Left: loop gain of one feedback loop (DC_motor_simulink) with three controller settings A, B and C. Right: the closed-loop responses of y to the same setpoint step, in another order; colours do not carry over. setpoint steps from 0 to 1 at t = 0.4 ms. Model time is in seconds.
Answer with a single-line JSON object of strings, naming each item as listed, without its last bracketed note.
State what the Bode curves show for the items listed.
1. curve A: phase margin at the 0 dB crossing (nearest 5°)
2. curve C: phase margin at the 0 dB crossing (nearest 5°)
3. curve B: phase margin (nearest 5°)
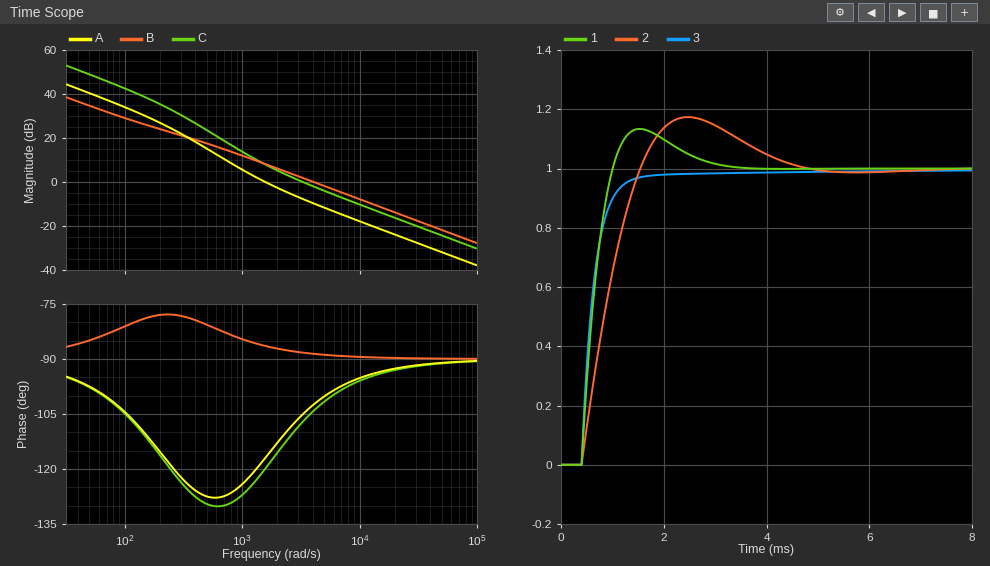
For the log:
{"curve A: phase margin at the 0 dB crossing": "65°", "curve C: phase margin at the 0 dB crossing": "75°", "curve B: phase margin": "90°"}
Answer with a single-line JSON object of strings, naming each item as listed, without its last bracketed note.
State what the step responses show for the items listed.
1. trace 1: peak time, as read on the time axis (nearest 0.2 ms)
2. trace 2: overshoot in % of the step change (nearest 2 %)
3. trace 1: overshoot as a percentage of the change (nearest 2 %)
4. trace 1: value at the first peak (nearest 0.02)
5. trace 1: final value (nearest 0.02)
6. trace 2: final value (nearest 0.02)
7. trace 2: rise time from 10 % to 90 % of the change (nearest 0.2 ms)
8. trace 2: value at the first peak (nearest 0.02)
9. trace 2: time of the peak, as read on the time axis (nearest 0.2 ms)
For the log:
{"trace 1: peak time, as read on the time axis": "1.6 ms", "trace 2: overshoot in % of the step change": "18 %", "trace 1: overshoot as a percentage of the change": "14 %", "trace 1: value at the first peak": "1.14", "trace 1: final value": "1.00", "trace 2: final value": "1.00", "trace 2: rise time from 10 % to 90 % of the change": "0.8 ms", "trace 2: value at the first peak": "1.18", "trace 2: time of the peak, as read on the time axis": "2.4 ms"}
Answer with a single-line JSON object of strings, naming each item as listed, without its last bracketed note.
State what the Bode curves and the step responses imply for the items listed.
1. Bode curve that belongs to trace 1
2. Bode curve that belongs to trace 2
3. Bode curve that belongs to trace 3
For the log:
{"Bode curve that belongs to trace 1": "C", "Bode curve that belongs to trace 2": "A", "Bode curve that belongs to trace 3": "B"}
